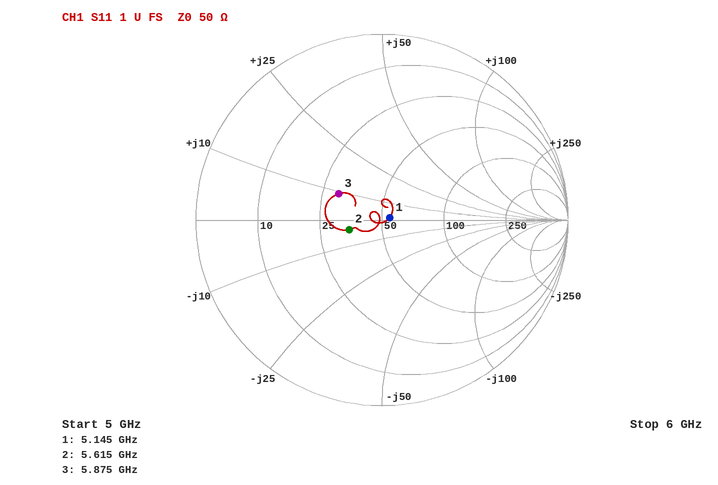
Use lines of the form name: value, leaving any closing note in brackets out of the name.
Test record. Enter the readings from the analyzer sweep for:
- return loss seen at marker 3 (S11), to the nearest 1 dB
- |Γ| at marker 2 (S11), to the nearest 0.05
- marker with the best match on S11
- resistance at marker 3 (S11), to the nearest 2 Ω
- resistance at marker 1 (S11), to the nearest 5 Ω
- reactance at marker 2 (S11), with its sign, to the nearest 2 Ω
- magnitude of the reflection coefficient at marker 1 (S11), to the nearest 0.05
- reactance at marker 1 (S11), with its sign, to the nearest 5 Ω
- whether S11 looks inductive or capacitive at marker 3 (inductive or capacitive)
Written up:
return loss seen at marker 3 (S11), to the nearest 1 dB: 11 dB
|Γ| at marker 2 (S11), to the nearest 0.05: 0.20
marker with the best match on S11: marker 1
resistance at marker 3 (S11), to the nearest 2 Ω: 30 Ω
resistance at marker 1 (S11), to the nearest 5 Ω: 55 Ω
reactance at marker 2 (S11), with its sign, to the nearest 2 Ω: -4 Ω
magnitude of the reflection coefficient at marker 1 (S11), to the nearest 0.05: 0.05
reactance at marker 1 (S11), with its sign, to the nearest 5 Ω: 0 Ω
whether S11 looks inductive or capacitive at marker 3: inductive
